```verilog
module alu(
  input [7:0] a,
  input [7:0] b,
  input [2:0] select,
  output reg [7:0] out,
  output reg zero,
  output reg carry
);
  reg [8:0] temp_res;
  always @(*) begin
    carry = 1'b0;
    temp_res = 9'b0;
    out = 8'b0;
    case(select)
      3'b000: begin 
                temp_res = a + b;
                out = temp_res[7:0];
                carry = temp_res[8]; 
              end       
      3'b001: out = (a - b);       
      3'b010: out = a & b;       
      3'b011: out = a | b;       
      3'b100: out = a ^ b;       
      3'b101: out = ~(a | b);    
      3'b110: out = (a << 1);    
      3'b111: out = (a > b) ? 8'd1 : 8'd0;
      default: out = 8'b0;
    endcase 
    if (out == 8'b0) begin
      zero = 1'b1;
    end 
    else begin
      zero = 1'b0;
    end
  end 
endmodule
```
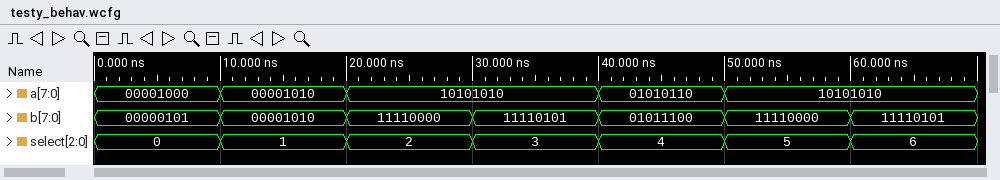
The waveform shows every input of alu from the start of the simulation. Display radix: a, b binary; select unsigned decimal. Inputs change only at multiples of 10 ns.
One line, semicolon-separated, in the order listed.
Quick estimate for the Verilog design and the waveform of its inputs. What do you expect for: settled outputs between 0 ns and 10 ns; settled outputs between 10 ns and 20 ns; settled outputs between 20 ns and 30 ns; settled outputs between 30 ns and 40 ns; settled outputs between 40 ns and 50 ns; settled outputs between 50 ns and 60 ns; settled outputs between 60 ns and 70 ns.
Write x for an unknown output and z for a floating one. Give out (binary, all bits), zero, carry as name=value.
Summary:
out=00001101, zero=0, carry=0; out=00000000, zero=1, carry=0; out=10100000, zero=0, carry=0; out=11111111, zero=0, carry=0; out=00001010, zero=0, carry=0; out=00000101, zero=0, carry=0; out=01010100, zero=0, carry=0
